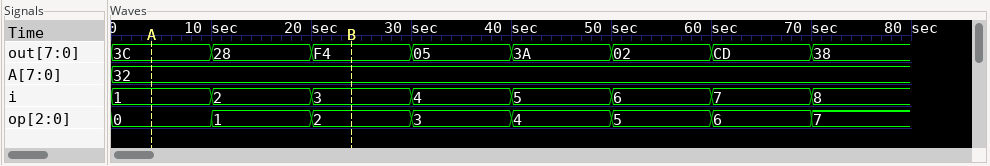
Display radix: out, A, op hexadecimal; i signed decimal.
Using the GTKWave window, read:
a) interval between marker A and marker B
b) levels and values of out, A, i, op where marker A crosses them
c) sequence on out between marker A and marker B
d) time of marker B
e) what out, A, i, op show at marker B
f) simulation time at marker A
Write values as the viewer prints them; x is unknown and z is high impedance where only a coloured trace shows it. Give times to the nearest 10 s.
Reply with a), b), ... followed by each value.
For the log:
a) 20 s
b) out=3C, A=32, i=1, op=0
c) 3C, 28, F4
d) 20 s
e) out=F4, A=32, i=3, op=2
f) 0 s
